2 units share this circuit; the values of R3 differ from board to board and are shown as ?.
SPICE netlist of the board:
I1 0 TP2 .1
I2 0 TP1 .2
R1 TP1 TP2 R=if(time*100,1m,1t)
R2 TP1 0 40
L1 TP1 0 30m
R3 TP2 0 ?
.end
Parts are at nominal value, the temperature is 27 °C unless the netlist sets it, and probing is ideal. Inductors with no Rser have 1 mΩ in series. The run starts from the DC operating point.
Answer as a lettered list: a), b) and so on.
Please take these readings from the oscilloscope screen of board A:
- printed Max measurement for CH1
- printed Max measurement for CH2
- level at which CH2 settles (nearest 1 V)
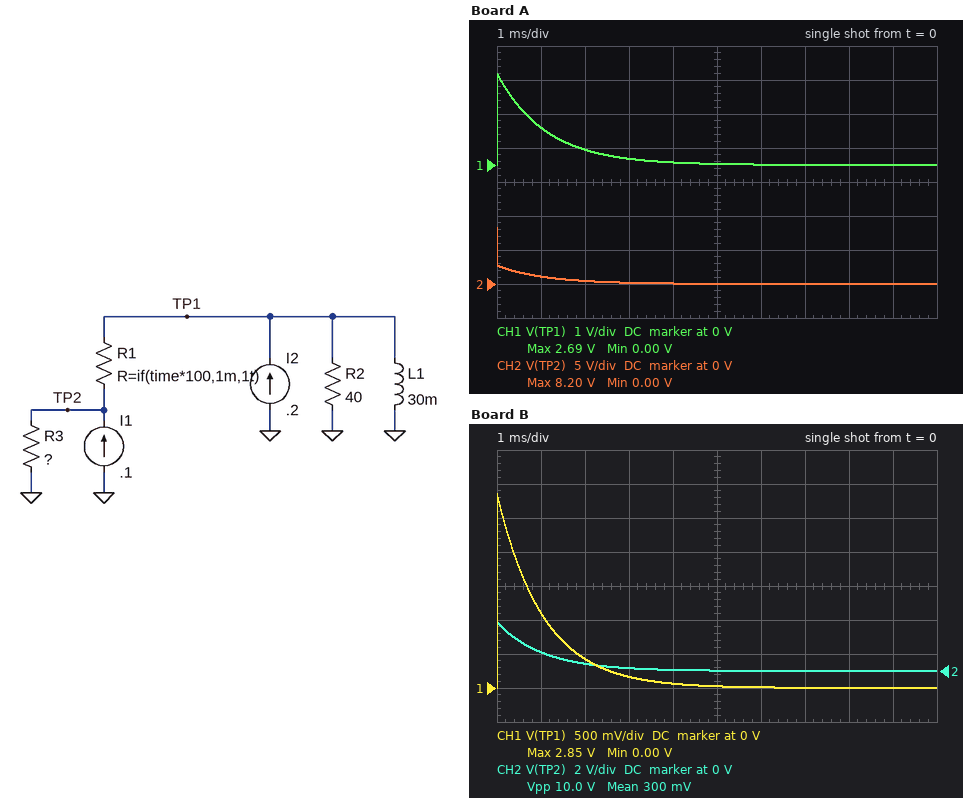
a) 2.69 V
b) 8.20 V
c) 0 V
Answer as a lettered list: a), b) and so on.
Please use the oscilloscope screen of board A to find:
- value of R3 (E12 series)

a) 82 Ω
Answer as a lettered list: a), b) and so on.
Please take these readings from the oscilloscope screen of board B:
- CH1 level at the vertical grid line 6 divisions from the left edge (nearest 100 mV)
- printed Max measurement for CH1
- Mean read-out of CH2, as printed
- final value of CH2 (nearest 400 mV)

a) 0 V
b) 2.85 V
c) 300 mV
d) 0 V
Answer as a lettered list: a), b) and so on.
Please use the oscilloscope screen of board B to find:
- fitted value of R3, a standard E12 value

a) 100 Ω
